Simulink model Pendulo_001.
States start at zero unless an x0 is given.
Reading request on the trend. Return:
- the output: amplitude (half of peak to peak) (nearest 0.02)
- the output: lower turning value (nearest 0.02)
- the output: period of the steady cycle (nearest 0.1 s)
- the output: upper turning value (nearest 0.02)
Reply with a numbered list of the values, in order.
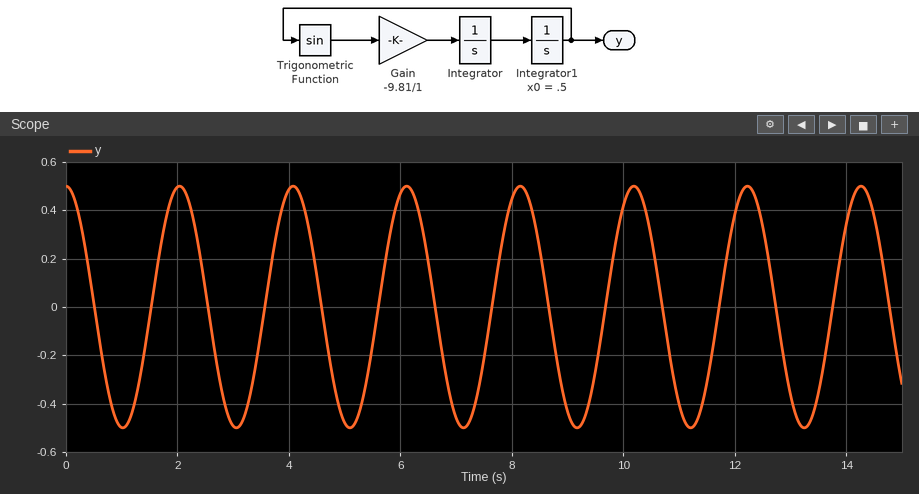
1. 0.50
2. -0.50
3. 2.0 s
4. 0.50
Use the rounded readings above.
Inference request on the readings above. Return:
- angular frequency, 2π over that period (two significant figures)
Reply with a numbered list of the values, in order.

1. 3.1 rad/s
